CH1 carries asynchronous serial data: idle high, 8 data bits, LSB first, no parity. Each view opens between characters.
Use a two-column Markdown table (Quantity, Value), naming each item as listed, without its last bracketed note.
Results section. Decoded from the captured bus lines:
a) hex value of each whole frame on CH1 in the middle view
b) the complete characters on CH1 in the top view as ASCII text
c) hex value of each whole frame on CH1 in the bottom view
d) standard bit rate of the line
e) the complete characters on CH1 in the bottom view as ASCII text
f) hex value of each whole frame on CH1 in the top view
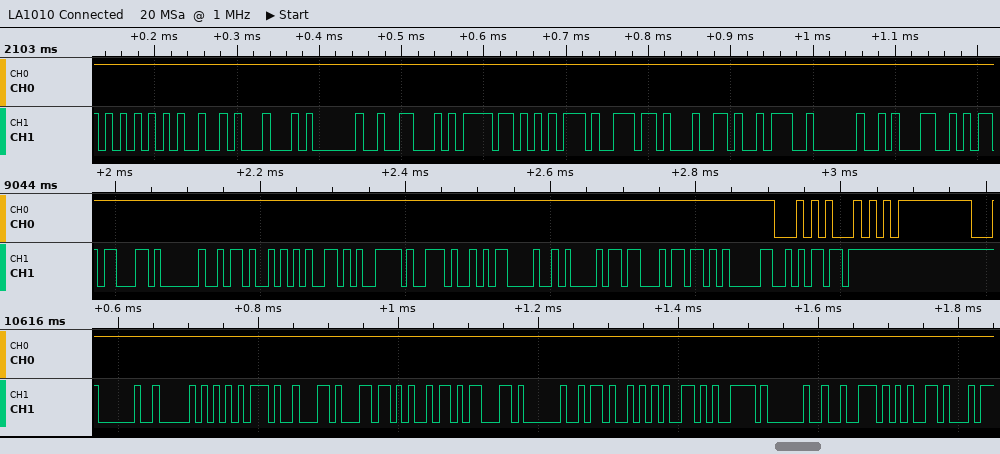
| Quantity | Value |
|---|---|
| hex value of each whole frame on CH1 in the middle view | 63, 20, 4B, 65, 79, 2E, 0D, 0A, 1B, 5B, 30, 6D |
| the complete characters on CH1 in the top view as ASCII text | "UID Found: 1" |
| hex value of each whole frame on CH1 in the bottom view | 20, 50, 75, 62, 6C, 69, 63, 20, 4B, 65, 79, 20, 72, 65 |
| standard bit rate of the line | 115200 baud |
| the complete characters on CH1 in the bottom view as ASCII text | " Public Key re" |
| hex value of each whole frame on CH1 in the top view | 55, 49, 44, 20, 46, 6F, 75, 6E, 64, 3A, 20, 31 |
